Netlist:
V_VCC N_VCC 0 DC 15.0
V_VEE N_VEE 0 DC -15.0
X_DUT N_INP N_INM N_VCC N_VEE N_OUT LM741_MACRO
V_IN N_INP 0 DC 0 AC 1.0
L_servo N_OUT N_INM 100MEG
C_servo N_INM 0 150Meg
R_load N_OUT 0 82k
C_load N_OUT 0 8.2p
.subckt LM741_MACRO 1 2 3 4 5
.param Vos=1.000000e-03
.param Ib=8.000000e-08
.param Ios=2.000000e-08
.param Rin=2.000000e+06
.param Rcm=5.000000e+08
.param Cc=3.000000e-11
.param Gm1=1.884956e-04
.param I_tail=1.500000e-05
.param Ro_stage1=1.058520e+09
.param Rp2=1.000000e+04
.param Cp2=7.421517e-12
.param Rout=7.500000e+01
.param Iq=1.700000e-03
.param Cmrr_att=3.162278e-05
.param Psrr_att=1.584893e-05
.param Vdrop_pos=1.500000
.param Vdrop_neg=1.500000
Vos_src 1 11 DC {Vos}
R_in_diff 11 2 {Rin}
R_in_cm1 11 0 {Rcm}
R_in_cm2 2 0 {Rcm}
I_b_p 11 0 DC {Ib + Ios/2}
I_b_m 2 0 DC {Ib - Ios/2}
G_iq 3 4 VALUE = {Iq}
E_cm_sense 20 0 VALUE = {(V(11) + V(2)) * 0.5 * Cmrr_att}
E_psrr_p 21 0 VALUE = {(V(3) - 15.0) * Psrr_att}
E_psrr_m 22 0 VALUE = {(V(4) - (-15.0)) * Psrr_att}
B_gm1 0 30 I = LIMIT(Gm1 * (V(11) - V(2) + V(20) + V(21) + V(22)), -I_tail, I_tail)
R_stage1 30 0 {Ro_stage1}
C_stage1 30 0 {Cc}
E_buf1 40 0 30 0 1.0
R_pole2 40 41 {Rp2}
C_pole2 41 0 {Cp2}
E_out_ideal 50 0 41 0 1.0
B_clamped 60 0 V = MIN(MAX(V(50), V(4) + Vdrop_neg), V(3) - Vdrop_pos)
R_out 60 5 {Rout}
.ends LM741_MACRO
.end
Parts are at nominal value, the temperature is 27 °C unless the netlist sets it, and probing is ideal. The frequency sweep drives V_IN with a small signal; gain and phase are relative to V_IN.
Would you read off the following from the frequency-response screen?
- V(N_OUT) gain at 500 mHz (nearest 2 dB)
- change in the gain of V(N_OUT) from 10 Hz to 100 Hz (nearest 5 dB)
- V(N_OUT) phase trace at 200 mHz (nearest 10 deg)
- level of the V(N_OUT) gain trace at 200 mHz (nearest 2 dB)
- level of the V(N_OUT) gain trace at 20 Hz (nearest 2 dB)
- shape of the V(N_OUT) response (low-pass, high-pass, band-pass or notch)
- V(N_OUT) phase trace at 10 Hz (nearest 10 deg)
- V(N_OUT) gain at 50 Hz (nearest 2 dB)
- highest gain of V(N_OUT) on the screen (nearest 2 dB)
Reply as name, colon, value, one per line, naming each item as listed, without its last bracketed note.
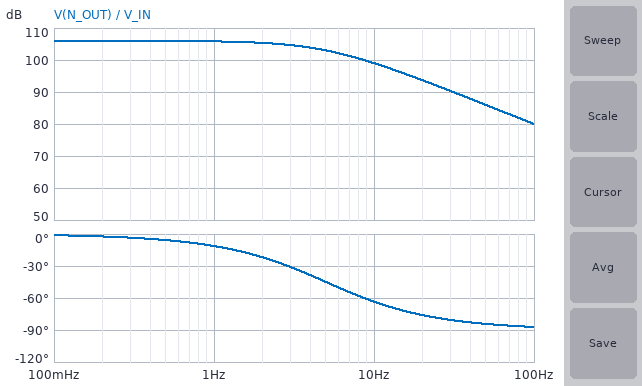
V(N_OUT) gain at 500 mHz: 106 dB
change in the gain of V(N_OUT) from 10 Hz to 100 Hz: -20 dB
V(N_OUT) phase trace at 200 mHz: 0 deg
level of the V(N_OUT) gain trace at 200 mHz: 106 dB
level of the V(N_OUT) gain trace at 20 Hz: 94 dB
shape of the V(N_OUT) response: low-pass
V(N_OUT) phase trace at 10 Hz: -60 deg
V(N_OUT) gain at 50 Hz: 86 dB
highest gain of V(N_OUT) on the screen: 106 dB
